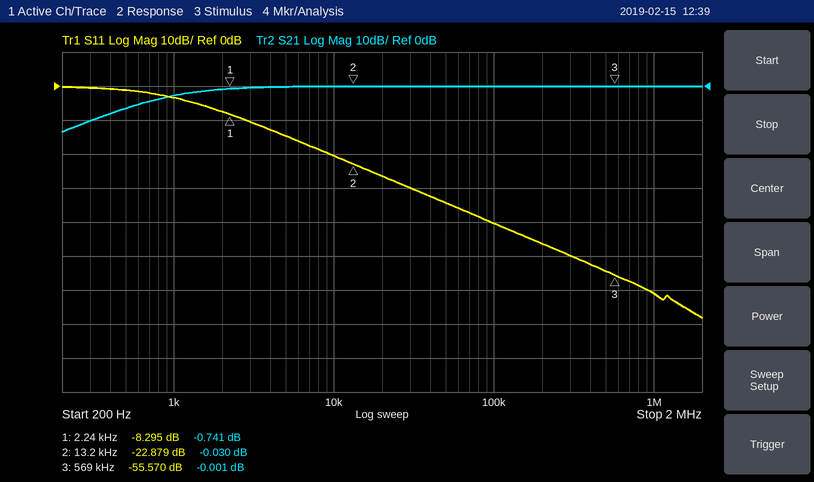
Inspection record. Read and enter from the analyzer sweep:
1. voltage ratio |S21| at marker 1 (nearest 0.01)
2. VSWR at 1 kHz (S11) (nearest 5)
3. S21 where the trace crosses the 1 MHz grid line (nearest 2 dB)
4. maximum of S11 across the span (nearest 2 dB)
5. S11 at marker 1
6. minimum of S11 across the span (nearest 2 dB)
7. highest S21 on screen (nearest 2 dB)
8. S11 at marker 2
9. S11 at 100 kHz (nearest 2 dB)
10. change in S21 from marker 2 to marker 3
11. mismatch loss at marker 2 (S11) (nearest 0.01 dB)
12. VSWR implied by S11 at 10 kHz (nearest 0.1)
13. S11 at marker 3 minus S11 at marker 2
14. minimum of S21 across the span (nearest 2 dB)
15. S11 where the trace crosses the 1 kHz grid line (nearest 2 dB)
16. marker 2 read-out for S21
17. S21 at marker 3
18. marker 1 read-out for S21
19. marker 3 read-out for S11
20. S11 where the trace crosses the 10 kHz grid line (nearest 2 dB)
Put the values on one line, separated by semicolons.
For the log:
0.92; 5; 0 dB; 0 dB; -8.295 dB; -68 dB; 0 dB; -22.879 dB; -40 dB; 0.029 dB; 0.02 dB; 1.2; -32.691 dB; -14 dB; -4 dB; -0.030 dB; -0.001 dB; -0.741 dB; -55.570 dB; -20 dB
